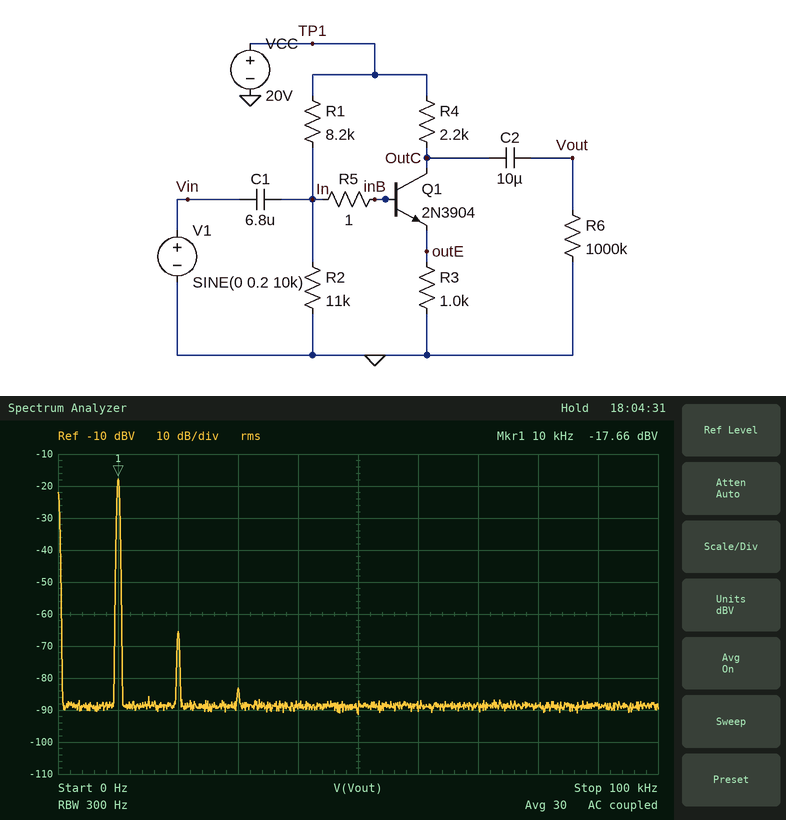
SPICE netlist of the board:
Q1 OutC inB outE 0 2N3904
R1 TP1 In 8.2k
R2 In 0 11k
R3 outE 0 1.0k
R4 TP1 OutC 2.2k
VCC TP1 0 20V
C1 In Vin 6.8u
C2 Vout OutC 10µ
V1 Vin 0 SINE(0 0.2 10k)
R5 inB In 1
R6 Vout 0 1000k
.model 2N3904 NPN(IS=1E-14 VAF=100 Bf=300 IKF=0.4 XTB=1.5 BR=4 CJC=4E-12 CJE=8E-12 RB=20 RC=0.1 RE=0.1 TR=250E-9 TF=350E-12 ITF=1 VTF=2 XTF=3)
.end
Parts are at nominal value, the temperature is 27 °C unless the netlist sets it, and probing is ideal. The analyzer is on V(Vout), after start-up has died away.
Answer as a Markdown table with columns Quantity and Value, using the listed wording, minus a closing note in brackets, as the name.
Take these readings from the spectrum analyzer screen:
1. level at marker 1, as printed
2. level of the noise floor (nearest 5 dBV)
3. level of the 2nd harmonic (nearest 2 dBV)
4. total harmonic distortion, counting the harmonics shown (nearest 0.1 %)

| Quantity | Value |
|---|---|
| level at marker 1, as printed | -17.66 dBV |
| level of the noise floor | -90 dBV |
| level of the 2nd harmonic | -66 dBV |
| total harmonic distortion, counting the harmonics shown | 0.4 % |
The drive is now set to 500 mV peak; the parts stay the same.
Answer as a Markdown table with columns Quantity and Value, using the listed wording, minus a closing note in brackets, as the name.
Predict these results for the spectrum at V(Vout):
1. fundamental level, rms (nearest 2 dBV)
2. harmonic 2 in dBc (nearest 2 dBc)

| Quantity | Value |
|---|---|
| fundamental level, rms | -10 dBV |
| harmonic 2 in dBc | -36 dBc |
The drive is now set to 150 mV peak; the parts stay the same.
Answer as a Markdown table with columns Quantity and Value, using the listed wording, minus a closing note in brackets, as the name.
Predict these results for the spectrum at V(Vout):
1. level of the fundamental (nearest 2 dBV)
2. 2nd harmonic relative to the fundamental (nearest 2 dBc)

| Quantity | Value |
|---|---|
| level of the fundamental | -20 dBV |
| 2nd harmonic relative to the fundamental | -50 dBc |
